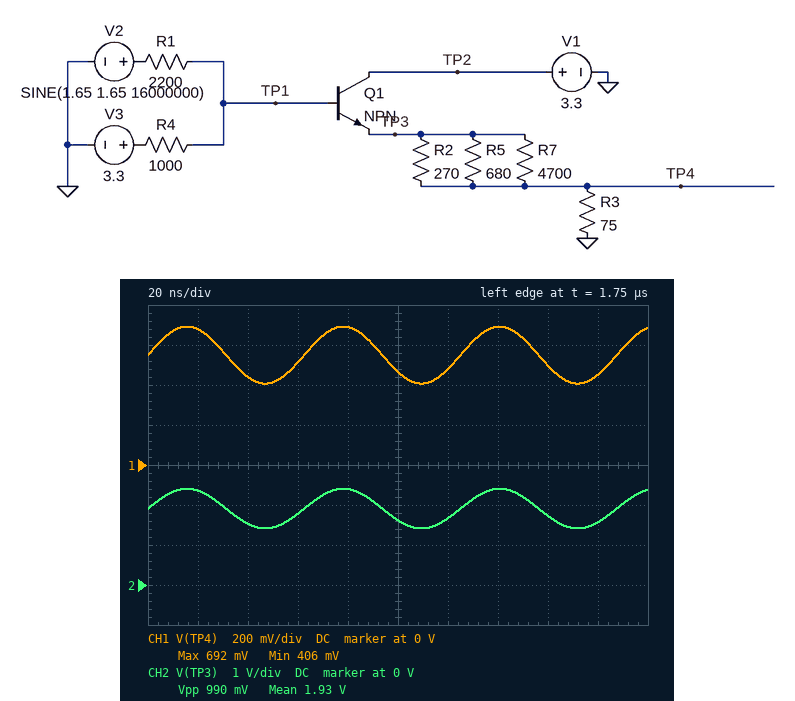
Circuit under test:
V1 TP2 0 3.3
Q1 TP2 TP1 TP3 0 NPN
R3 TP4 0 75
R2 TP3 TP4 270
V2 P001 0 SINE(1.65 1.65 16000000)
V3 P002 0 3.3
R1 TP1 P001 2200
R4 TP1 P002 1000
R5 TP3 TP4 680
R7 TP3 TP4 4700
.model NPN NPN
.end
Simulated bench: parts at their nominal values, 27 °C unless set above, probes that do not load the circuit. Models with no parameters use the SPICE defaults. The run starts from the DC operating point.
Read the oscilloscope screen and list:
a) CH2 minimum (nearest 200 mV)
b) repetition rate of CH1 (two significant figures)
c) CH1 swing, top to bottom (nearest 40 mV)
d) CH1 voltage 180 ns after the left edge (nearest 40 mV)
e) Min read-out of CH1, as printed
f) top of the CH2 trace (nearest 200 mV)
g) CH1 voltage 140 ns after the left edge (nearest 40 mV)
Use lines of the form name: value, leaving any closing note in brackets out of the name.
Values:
CH2 minimum: 1.4 V
repetition rate of CH1: 16 MHz
CH1 swing, top to bottom: 280 mV
CH1 voltage 180 ns after the left edge: 440 mV
Min read-out of CH1, as printed: 406 mV
top of the CH2 trace: 2.4 V
CH1 voltage 140 ns after the left edge: 680 mV
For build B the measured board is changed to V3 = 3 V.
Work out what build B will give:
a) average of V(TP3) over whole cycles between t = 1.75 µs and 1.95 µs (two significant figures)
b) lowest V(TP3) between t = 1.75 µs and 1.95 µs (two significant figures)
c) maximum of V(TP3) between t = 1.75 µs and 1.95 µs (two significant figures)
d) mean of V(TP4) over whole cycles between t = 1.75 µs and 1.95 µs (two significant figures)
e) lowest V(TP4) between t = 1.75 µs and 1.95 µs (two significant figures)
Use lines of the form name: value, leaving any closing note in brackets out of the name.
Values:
average of V(TP3) over whole cycles between t = 1.75 µs and 1.95 µs: 1.7 V
lowest V(TP3) between t = 1.75 µs and 1.95 µs: 1.2 V
maximum of V(TP3) between t = 1.75 µs and 1.95 µs: 2.2 V
mean of V(TP4) over whole cycles between t = 1.75 µs and 1.95 µs: 490 mV
lowest V(TP4) between t = 1.75 µs and 1.95 µs: 350 mV
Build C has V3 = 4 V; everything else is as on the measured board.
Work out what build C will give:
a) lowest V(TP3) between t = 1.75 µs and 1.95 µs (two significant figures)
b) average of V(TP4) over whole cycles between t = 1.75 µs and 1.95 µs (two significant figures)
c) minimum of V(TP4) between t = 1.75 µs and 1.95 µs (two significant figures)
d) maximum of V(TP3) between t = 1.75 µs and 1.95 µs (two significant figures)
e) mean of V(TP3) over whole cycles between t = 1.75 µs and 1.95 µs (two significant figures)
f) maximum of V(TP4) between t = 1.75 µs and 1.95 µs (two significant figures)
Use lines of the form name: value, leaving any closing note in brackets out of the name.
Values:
lowest V(TP3) between t = 1.75 µs and 1.95 µs: 1.9 V
average of V(TP4) over whole cycles between t = 1.75 µs and 1.95 µs: 680 mV
minimum of V(TP4) between t = 1.75 µs and 1.95 µs: 540 mV
maximum of V(TP3) between t = 1.75 µs and 1.95 µs: 2.9 V
mean of V(TP3) over whole cycles between t = 1.75 µs and 1.95 µs: 2.4 V
maximum of V(TP4) between t = 1.75 µs and 1.95 µs: 830 mV
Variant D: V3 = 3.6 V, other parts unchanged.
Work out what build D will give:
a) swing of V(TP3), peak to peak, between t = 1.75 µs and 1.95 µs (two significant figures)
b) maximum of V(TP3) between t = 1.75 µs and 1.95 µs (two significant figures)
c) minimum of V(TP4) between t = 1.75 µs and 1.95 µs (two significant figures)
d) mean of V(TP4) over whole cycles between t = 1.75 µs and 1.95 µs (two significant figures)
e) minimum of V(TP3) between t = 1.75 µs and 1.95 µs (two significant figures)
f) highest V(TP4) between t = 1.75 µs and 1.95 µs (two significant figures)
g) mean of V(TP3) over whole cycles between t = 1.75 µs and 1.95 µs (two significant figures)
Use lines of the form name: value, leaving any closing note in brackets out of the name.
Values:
swing of V(TP3), peak to peak, between t = 1.75 µs and 1.95 µs: 990 mV
maximum of V(TP3) between t = 1.75 µs and 1.95 µs: 2.6 V
minimum of V(TP4) between t = 1.75 µs and 1.95 µs: 460 mV
mean of V(TP4) over whole cycles between t = 1.75 µs and 1.95 µs: 610 mV
minimum of V(TP3) between t = 1.75 µs and 1.95 µs: 1.6 V
highest V(TP4) between t = 1.75 µs and 1.95 µs: 750 mV
mean of V(TP3) over whole cycles between t = 1.75 µs and 1.95 µs: 2.1 V
